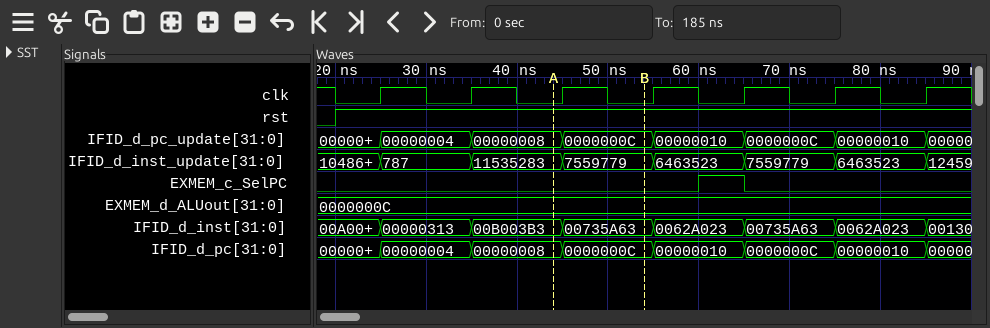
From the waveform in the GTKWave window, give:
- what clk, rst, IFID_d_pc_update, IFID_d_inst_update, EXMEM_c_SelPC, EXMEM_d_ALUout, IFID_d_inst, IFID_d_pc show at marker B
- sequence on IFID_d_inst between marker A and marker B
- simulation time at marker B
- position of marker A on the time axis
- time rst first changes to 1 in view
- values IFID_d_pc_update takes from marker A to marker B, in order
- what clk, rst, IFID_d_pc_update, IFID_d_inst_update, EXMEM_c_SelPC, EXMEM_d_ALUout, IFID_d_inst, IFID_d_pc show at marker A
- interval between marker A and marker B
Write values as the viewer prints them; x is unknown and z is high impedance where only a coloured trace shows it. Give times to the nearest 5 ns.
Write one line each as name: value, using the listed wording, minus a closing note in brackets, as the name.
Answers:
what clk, rst, IFID_d_pc_update, IFID_d_inst_update, EXMEM_c_SelPC, EXMEM_d_ALUout, IFID_d_inst, IFID_d_pc show at marker B: clk=0, rst=1, IFID_d_pc_update=0000000C, IFID_d_inst_update=7559779, EXMEM_c_SelPC=0, EXMEM_d_ALUout=0000000C, IFID_d_inst=00735A63, IFID_d_pc=0000000C
sequence on IFID_d_inst between marker A and marker B: 00B003B3, 00735A63
simulation time at marker B: 55 ns
position of marker A on the time axis: 45 ns
time rst first changes to 1 in view: 20 ns
values IFID_d_pc_update takes from marker A to marker B, in order: 00000008, 0000000C
what clk, rst, IFID_d_pc_update, IFID_d_inst_update, EXMEM_c_SelPC, EXMEM_d_ALUout, IFID_d_inst, IFID_d_pc show at marker A: clk=0, rst=1, IFID_d_pc_update=00000008, IFID_d_inst_update=11535283, EXMEM_c_SelPC=0, EXMEM_d_ALUout=0000000C, IFID_d_inst=00B003B3, IFID_d_pc=00000008
interval between marker A and marker B: 10 ns
